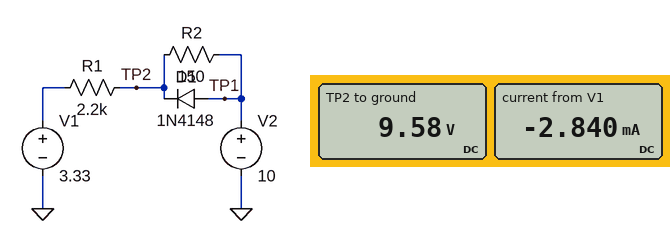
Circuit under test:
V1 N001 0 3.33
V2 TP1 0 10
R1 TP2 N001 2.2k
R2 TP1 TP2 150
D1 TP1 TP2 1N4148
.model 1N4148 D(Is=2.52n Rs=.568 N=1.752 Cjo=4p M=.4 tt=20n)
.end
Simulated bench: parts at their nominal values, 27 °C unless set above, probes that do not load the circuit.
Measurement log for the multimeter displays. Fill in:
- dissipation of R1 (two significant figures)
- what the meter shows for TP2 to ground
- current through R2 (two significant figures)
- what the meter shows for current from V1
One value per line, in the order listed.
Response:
18 mW
9.58 V
2.8 mA
-2.840 mA
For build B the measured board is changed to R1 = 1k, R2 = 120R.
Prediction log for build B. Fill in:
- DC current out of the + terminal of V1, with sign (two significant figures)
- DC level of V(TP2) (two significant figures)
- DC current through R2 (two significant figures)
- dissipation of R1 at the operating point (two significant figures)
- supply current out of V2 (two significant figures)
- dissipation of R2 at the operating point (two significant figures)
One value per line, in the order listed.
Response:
-6.1 mA
9.4 V
4.9 mA
37 mW
6.1 mA
2.9 mW
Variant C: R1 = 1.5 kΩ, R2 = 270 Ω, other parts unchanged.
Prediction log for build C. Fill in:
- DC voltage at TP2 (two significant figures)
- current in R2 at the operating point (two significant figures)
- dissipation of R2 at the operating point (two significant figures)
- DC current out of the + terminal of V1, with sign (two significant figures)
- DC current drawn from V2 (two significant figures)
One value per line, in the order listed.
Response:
9.4 V
2.3 mA
1.4 mW
-4.0 mA
4.0 mA
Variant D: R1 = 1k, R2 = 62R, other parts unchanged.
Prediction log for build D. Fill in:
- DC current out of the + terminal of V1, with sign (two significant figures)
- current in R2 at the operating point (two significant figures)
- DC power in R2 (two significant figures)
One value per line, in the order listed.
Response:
-6.3 mA
6.3 mA
2.4 mW
